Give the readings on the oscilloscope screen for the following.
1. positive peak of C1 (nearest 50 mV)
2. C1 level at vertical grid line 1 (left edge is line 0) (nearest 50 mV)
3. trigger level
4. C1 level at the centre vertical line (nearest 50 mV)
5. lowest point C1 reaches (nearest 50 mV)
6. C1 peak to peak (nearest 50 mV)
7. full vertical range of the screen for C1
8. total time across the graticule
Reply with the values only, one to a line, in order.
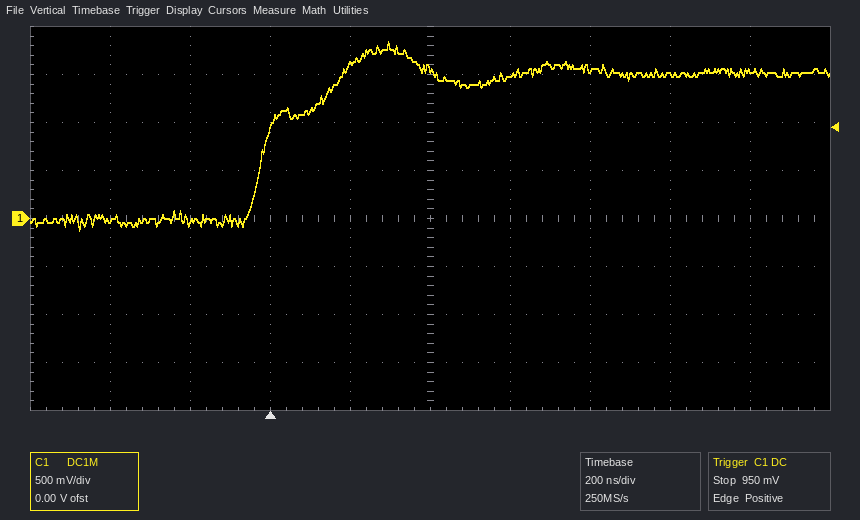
1.85 V
0 mV
950 mV
1.55 V
-100 mV
1.95 V
4 V
2 µs
